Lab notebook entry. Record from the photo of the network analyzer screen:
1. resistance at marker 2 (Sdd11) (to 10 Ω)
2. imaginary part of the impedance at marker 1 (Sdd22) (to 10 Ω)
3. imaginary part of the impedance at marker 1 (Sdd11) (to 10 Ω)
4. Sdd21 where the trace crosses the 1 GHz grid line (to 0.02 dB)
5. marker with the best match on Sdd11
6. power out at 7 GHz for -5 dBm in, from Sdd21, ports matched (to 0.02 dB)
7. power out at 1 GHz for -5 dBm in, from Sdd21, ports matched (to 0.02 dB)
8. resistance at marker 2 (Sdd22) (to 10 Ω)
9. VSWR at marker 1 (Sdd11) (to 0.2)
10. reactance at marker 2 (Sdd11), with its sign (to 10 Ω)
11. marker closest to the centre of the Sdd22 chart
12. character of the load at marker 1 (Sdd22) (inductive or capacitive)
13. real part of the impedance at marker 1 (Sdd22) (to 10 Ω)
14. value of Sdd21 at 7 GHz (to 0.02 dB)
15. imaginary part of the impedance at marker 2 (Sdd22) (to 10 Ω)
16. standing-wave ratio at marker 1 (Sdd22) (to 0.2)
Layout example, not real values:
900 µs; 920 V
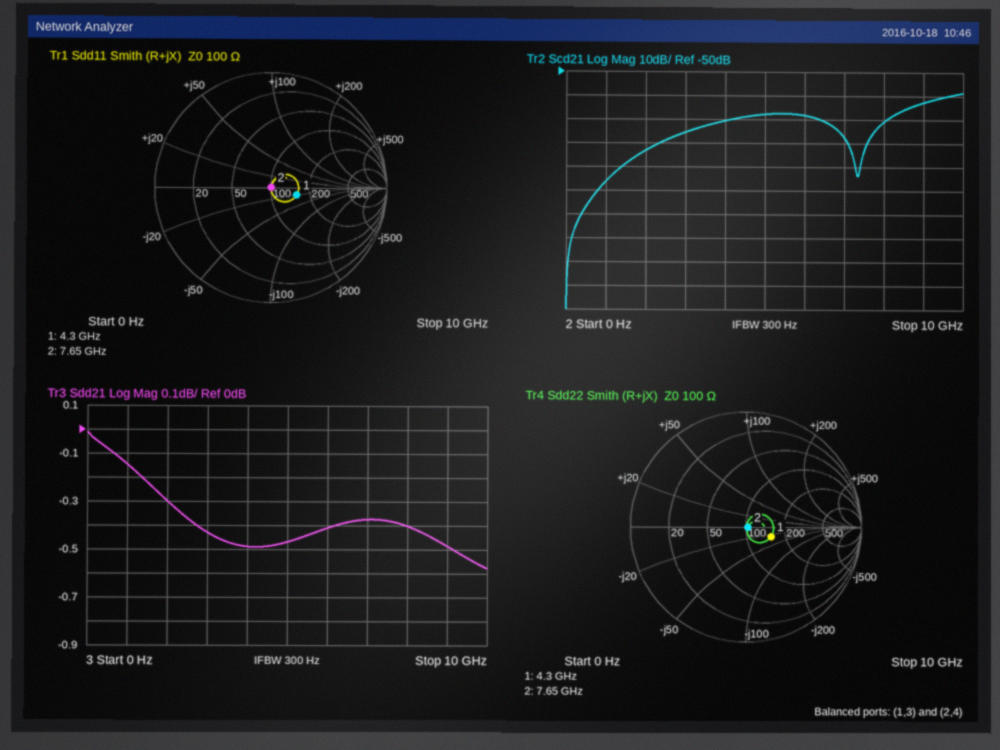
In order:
100 Ω; -30 Ω; -20 Ω; -0.14 dB; marker 2; -5.38 dBm; -5.14 dBm; 100 Ω; 1.6; 0 Ω; marker 2; capacitive; 150 Ω; -0.38 dB; 0 Ω; 1.6
